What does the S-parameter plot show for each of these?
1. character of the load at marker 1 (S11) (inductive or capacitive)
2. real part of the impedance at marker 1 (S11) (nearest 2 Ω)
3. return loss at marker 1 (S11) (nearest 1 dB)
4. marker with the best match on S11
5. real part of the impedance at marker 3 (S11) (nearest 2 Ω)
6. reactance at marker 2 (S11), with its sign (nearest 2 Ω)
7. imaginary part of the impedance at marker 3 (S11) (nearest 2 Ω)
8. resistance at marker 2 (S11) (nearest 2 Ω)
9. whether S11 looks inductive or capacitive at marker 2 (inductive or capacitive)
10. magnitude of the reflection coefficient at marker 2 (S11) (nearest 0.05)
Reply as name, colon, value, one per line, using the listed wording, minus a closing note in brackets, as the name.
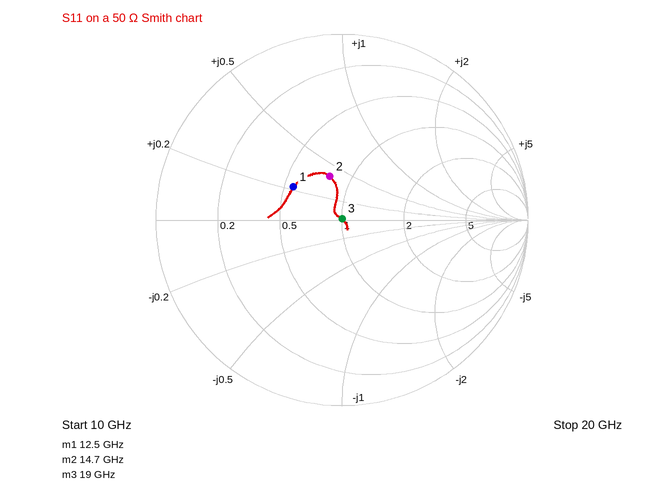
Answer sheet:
character of the load at marker 1 (S11): inductive
real part of the impedance at marker 1 (S11): 28 Ω
return loss at marker 1 (S11): 10 dB
marker with the best match on S11: marker 3
real part of the impedance at marker 3 (S11): 50 Ω
reactance at marker 2 (S11), with its sign: +20 Ω
imaginary part of the impedance at marker 3 (S11): 0 Ω
resistance at marker 2 (S11): 40 Ω
whether S11 looks inductive or capacitive at marker 2: inductive
magnitude of the reflection coefficient at marker 2 (S11): 0.25
